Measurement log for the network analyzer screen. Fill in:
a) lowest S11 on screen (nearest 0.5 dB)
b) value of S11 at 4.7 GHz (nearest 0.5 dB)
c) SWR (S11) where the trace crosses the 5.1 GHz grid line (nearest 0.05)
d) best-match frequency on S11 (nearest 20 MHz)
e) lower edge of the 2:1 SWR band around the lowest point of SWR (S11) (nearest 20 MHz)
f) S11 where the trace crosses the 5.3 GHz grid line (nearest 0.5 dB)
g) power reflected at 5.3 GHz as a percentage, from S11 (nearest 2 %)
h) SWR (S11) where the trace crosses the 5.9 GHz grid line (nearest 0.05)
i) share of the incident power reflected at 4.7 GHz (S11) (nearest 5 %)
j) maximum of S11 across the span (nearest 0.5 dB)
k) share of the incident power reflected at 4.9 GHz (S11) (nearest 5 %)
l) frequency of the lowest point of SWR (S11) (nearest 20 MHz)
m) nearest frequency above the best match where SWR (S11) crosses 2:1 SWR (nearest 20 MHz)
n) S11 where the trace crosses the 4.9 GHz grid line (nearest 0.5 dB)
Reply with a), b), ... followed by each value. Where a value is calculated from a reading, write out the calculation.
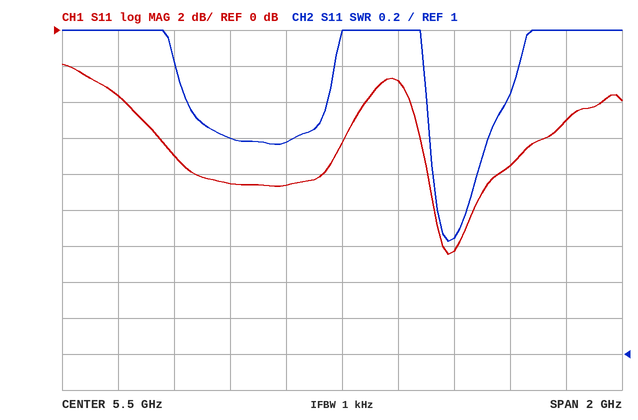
a) -12.5 dB
b) -3.5 dB
c) 2.20
d) 5.88 GHz
e) 5.82 GHz
f) -8.5 dB
g) 10^(-8.5/10) ≈ 14 %
h) 1.65
i) 10^(-3.5/10) ≈ 45 %
j) -2.0 dB
k) 10^(-7/10) ≈ 20 %
l) 5.88 GHz
m) 5.98 GHz
n) -7.0 dB
